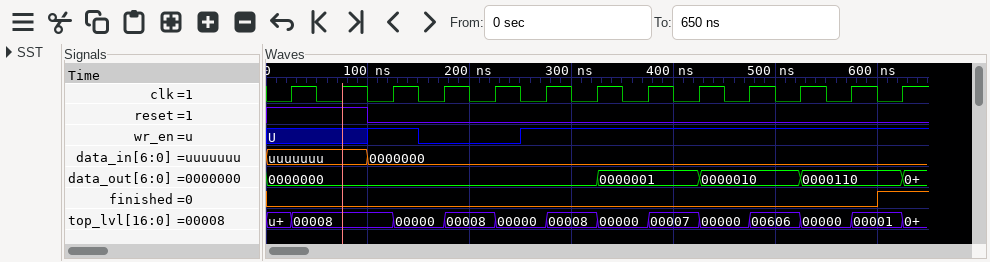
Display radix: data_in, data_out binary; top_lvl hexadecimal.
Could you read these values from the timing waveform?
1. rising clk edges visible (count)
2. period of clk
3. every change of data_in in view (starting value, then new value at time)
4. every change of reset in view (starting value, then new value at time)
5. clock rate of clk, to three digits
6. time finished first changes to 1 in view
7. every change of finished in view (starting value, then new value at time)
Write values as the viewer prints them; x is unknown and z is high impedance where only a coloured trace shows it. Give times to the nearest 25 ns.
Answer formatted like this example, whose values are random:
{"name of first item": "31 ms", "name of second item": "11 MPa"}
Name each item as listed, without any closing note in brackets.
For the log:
{"rising clk edges visible": "13", "period of clk": "50 ns", "every change of data_in in view": "uuuuuuu, 0000000 at 100 ns", "every change of reset in view": "1, 0 at 100 ns", "clock rate of clk, to three digits": "20.0 MHz", "time finished first changes to 1 in view": "600 ns", "every change of finished in view": "0, 1 at 600 ns"}
